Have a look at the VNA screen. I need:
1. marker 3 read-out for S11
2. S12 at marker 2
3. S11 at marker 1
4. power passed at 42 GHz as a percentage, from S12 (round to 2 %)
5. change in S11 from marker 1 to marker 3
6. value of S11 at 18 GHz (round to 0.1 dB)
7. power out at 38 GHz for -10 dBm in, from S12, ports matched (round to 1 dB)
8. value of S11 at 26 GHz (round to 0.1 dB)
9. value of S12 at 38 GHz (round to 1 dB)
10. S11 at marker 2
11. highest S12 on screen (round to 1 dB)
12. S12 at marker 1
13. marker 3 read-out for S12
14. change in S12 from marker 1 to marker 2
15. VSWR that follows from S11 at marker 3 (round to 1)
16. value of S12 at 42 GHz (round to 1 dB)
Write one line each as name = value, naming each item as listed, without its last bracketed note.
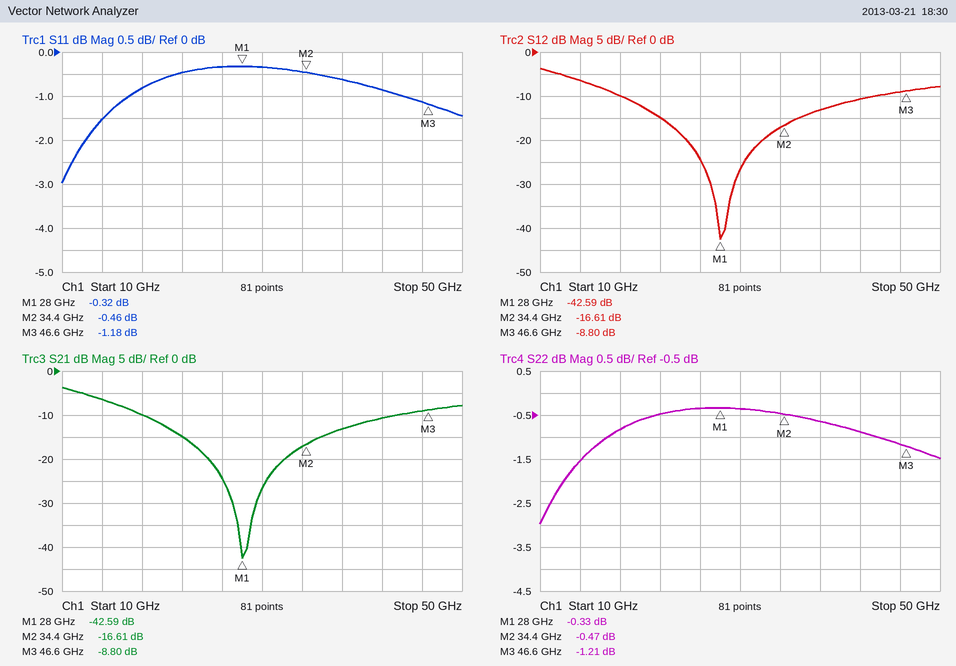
marker 3 read-out for S11 = -1.18 dB
S12 at marker 2 = -16.61 dB
S11 at marker 1 = -0.32 dB
power passed at 42 GHz as a percentage, from S12 = 8 %
change in S11 from marker 1 to marker 3 = -0.86 dB
value of S11 at 18 GHz = -0.8 dB
power out at 38 GHz for -10 dBm in, from S12, ports matched = -23 dBm
value of S11 at 26 GHz = -0.3 dB
value of S12 at 38 GHz = -13 dB
S11 at marker 2 = -0.46 dB
highest S12 on screen = -4 dB
S12 at marker 1 = -42.59 dB
marker 3 read-out for S12 = -8.80 dB
change in S12 from marker 1 to marker 2 = 25.98 dB
VSWR that follows from S11 at marker 3 = 15
value of S12 at 42 GHz = -11 dB
